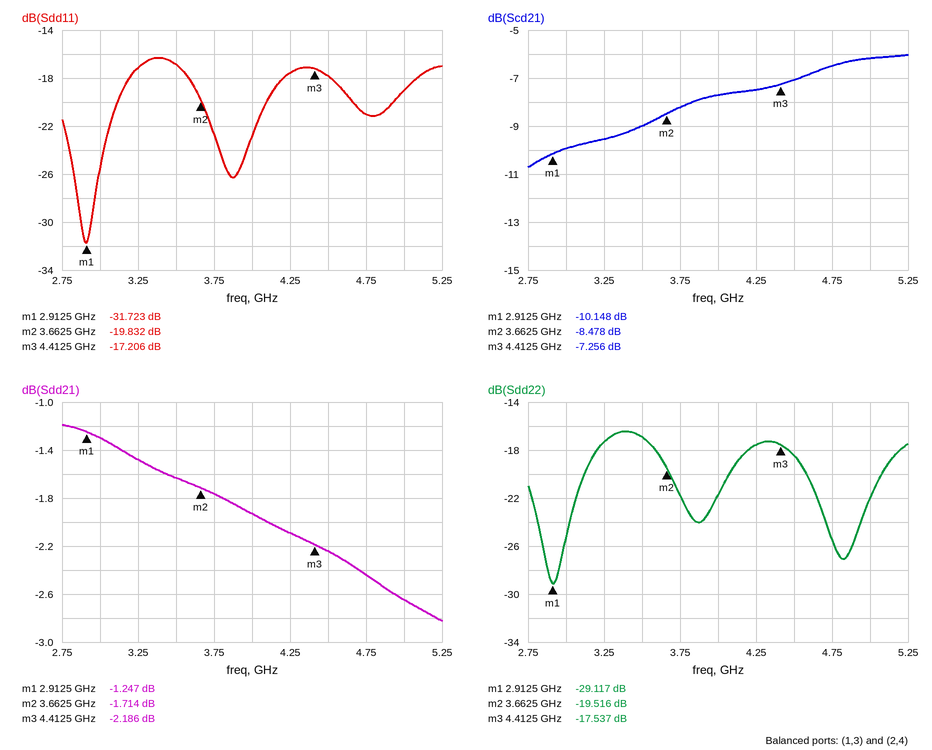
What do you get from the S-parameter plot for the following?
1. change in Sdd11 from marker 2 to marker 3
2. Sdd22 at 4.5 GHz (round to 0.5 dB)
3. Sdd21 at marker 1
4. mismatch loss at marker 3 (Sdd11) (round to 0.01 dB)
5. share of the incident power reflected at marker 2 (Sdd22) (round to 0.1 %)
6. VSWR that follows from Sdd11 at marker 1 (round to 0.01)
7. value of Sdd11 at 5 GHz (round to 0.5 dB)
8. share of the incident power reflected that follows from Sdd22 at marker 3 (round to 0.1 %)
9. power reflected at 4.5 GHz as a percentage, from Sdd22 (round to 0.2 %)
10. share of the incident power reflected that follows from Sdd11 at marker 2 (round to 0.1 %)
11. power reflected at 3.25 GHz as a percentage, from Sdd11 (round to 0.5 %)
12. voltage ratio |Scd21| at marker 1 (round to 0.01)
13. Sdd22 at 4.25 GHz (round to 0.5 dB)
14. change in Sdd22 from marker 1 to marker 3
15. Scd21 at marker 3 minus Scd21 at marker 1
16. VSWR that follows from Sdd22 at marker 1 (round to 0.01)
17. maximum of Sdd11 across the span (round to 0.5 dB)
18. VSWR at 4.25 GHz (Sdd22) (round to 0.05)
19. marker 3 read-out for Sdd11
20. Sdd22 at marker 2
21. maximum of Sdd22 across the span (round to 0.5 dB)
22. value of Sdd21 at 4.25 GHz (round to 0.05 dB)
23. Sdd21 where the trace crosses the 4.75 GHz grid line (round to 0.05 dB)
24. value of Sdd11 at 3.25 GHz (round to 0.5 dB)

2.626 dB
-18.5 dB
-1.247 dB
0.08 dB
1.1 %
1.05
-19.0 dB
1.8 %
1.4 %
1.0 %
2.0 %
0.31
-17.5 dB
11.580 dB
2.892 dB
1.07
-16.5 dB
1.30
-17.206 dB
-19.516 dB
-16.5 dB
-2.10 dB
-2.45 dB
-17.0 dB
